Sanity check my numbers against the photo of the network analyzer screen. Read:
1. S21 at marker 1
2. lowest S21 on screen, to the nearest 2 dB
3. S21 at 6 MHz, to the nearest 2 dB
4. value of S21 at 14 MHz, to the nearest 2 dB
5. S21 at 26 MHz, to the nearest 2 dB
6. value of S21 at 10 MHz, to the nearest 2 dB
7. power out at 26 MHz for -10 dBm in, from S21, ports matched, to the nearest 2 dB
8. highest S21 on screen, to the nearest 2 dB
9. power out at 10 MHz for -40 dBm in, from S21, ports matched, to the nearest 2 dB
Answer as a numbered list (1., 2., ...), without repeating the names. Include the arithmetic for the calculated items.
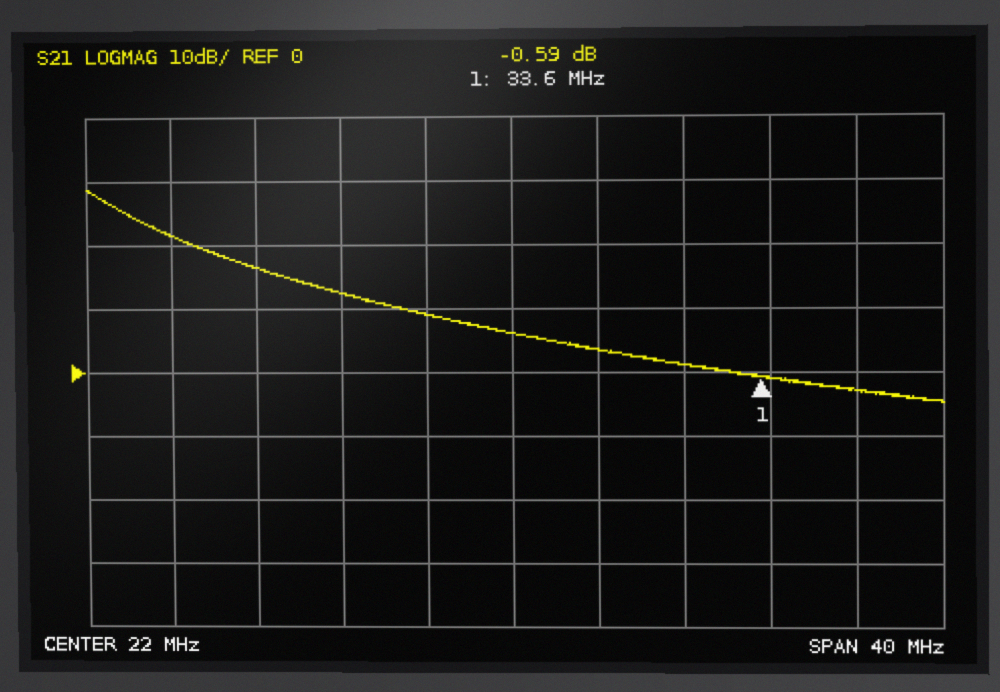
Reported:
1. -0.59 dB
2. -4 dB
3. 22 dB
4. 12 dB
5. 4 dB
6. 16 dB
7. -10 dBm + (4 dB) = -6 dBm
8. 28 dB
9. -40 dBm + (16 dB) = -24 dBm
